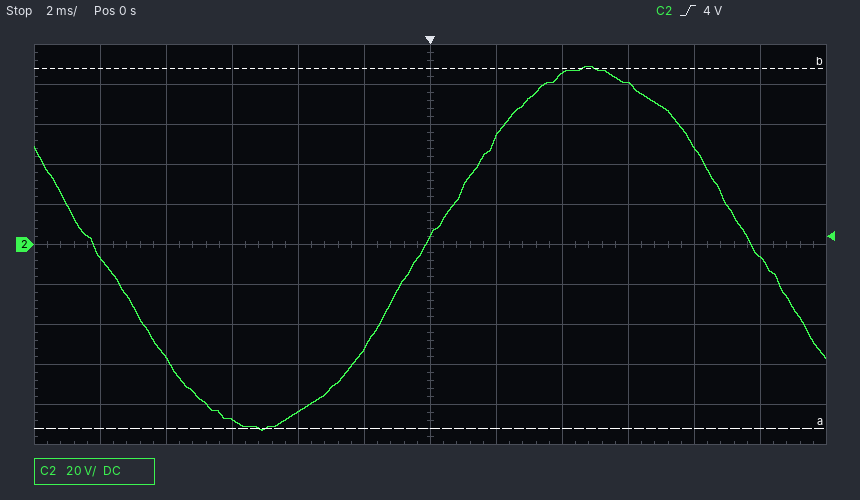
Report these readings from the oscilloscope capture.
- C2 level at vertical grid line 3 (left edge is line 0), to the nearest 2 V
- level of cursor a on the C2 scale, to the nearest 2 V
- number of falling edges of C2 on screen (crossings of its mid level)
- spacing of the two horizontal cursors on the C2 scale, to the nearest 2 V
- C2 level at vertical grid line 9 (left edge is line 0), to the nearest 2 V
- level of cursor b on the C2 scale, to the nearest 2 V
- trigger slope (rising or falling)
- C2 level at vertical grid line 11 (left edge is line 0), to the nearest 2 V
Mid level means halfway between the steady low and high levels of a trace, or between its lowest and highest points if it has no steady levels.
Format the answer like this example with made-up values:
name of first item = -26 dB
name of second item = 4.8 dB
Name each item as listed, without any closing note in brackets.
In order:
C2 level at vertical grid line 3 (left edge is line 0), to the nearest 2 V = -88 V
level of cursor a on the C2 scale, to the nearest 2 V = -92 V
number of falling edges of C2 on screen = 2
spacing of the two horizontal cursors on the C2 scale, to the nearest 2 V = 180 V
C2 level at vertical grid line 9 (left edge is line 0), to the nearest 2 V = 80 V
level of cursor b on the C2 scale, to the nearest 2 V = 88 V
trigger slope = rising
C2 level at vertical grid line 11 (left edge is line 0), to the nearest 2 V = -6 V
